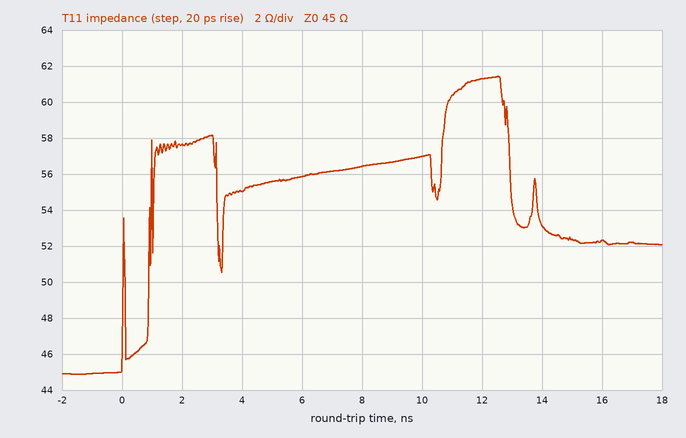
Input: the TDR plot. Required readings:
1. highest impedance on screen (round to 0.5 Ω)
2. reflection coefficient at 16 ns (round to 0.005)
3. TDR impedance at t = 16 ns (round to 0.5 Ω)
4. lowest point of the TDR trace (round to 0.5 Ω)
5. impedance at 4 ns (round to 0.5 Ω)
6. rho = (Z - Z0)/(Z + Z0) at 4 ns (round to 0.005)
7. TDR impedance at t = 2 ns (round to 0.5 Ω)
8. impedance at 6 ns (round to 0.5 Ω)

61.5 Ω
+0.075
52.5 Ω
45.0 Ω
55.0 Ω
+0.100
57.5 Ω
56.0 Ω
